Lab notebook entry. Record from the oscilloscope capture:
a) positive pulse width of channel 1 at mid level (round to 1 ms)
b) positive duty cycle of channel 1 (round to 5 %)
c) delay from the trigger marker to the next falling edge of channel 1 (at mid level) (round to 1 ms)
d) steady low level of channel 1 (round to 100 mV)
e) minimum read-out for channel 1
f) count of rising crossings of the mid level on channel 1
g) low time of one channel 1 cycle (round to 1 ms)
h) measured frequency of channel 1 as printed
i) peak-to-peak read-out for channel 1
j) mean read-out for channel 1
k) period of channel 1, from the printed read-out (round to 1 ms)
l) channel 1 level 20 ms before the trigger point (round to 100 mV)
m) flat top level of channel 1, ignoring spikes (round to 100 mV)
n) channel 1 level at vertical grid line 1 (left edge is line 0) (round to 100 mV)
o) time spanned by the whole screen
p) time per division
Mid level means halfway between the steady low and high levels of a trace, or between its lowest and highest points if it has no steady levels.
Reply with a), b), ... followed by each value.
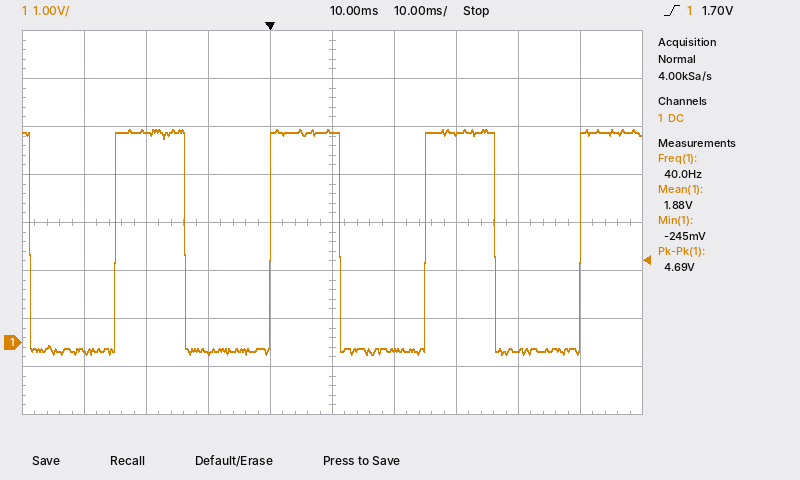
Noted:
a) 11 ms
b) 45 %
c) 11 ms
d) -200 mV
e) -245 mV
f) 4
g) 14 ms
h) 40.0 Hz
i) 4.69 V
j) 1.88 V
k) 25 ms
l) 4.4 V
m) 4.4 V
n) -200 mV
o) 100 ms
p) 10 ms
